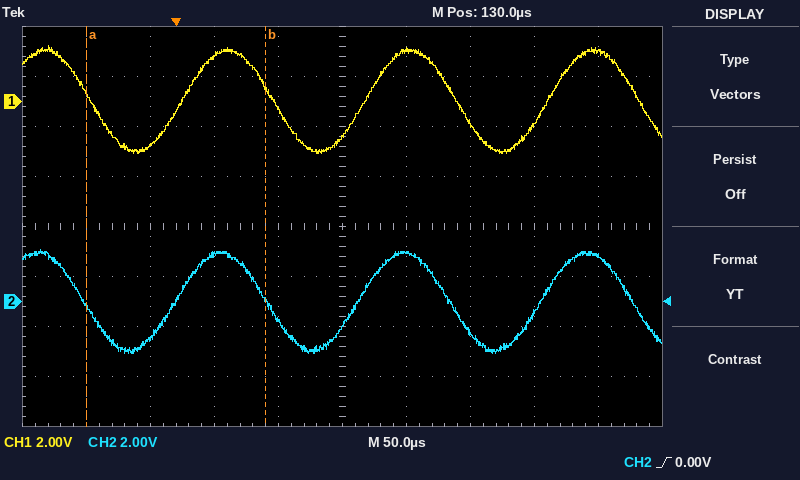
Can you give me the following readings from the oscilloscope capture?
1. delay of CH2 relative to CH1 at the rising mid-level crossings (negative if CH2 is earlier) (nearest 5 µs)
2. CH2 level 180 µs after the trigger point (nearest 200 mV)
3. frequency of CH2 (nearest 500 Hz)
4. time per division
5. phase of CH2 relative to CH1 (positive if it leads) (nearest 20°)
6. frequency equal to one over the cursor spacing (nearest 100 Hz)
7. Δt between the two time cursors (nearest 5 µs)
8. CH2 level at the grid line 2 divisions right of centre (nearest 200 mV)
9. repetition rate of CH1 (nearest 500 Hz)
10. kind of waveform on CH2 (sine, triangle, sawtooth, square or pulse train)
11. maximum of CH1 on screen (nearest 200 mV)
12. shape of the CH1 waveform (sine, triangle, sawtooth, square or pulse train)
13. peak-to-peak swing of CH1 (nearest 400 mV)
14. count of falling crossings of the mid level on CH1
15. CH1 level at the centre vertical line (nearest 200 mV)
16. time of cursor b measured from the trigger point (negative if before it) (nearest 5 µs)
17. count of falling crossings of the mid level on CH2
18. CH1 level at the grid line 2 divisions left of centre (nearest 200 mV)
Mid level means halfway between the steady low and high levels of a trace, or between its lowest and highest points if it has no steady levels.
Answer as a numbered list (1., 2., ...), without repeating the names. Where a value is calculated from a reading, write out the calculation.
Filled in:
1. -5 µs
2. 2.0 V
3. 7.0 kHz
4. 50 µs
5. +20°
6. 1 / 140 µs ≈ 7.1 kHz
7. 140 µs
8. -1.2 V
9. 7.0 kHz
10. sine
11. 2.2 V
12. sine
13. 4.4 V
14. 4
15. -1.4 V
16. +70 µs
17. 4
18. 1.8 V
